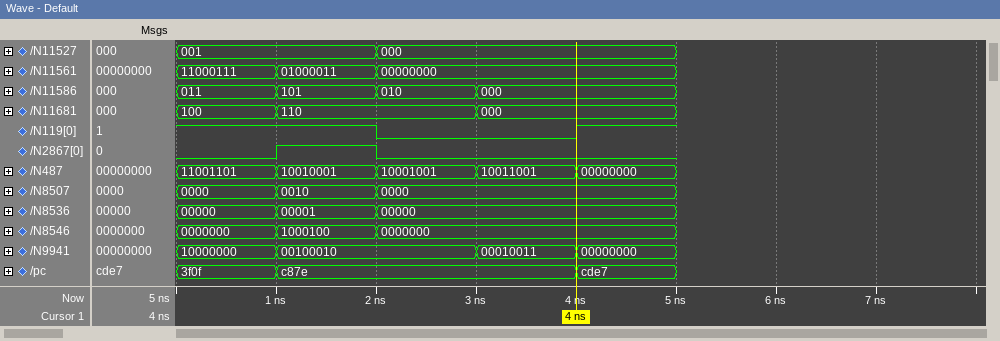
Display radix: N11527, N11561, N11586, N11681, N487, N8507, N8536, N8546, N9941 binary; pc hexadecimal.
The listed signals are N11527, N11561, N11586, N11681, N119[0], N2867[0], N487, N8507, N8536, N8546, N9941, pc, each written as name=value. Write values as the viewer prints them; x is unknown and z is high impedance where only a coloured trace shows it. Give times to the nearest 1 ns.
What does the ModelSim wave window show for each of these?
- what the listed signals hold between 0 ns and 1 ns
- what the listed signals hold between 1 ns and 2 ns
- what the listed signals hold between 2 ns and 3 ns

N11527=001, N11561=11000111, N11586=011, N11681=100, N119[0]=1, N2867[0]=0, N487=11001101, N8507=0000, N8536=00000, N8546=0000000, N9941=10000000, pc=3f0f
N11527=001, N11561=01000011, N11586=101, N11681=110, N119[0]=1, N2867[0]=1, N487=10010001, N8507=0010, N8536=00001, N8546=1000100, N9941=00100010, pc=c87e
N11527=000, N11561=00000000, N11586=010, N11681=110, N119[0]=0, N2867[0]=0, N487=10001001, N8507=0000, N8536=00000, N8546=0000000, N9941=00100010, pc=c87e
